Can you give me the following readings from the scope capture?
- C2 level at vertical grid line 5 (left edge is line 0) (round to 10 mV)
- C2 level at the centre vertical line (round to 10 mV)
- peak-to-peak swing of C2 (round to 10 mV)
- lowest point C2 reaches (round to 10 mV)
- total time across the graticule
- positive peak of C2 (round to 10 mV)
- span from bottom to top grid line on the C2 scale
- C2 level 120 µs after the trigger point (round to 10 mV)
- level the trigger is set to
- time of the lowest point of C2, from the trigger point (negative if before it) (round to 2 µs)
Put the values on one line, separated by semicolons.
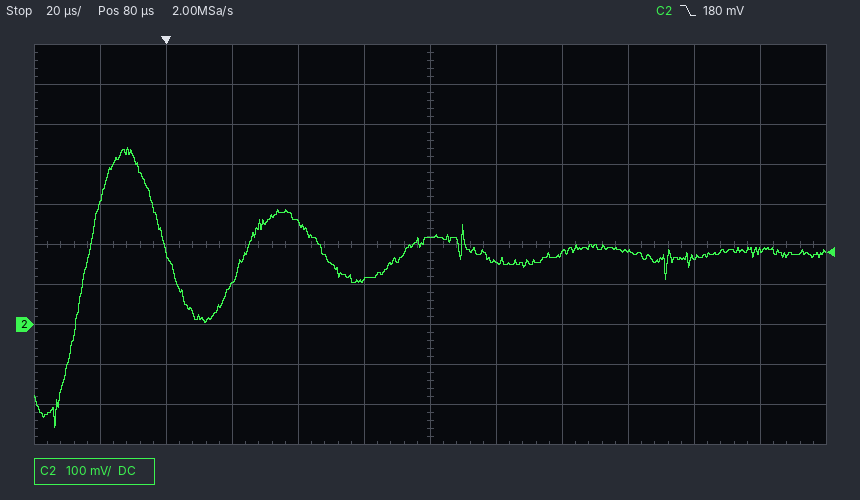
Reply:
110 mV; 220 mV; 700 mV; -260 mV; 240 µs; 440 mV; 1 V; 180 mV; 180 mV; -34 µs
